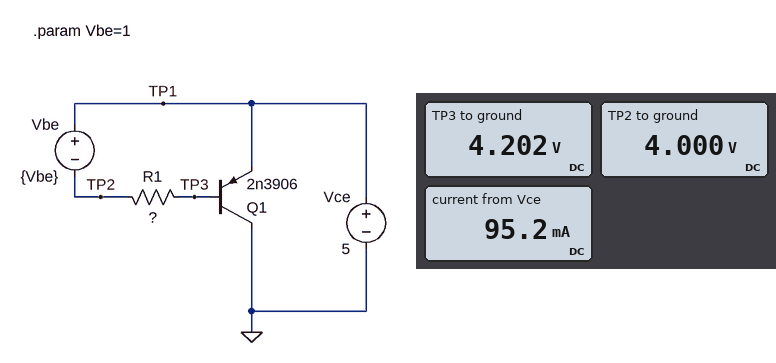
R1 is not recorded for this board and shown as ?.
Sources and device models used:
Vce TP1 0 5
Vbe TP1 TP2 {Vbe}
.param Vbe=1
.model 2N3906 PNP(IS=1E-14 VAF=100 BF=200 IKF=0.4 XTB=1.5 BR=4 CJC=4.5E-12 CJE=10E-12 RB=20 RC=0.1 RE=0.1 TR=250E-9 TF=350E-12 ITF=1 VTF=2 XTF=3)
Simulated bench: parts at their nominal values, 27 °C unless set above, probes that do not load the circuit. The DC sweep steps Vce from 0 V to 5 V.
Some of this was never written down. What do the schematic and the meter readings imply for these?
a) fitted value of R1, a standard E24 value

360 Ω
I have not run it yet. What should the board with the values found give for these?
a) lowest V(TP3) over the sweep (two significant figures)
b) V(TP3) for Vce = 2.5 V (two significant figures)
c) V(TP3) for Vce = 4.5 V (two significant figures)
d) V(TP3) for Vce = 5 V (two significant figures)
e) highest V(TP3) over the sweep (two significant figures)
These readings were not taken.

-700 mV
1.7 V
3.7 V
4.2 V
4.2 V
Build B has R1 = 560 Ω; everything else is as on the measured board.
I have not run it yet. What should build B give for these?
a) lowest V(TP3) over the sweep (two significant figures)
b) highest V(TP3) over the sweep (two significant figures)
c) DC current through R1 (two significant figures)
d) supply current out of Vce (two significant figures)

-690 mV
4.2 V
390 µA
69 mA
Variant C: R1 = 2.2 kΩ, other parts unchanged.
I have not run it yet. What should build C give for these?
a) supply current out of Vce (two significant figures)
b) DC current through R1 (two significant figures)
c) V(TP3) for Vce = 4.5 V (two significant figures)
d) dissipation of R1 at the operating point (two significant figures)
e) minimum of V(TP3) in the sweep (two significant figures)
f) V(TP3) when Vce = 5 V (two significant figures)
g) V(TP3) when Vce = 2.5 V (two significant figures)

23 mA
120 µA
3.8 V
30 µW
-650 mV
4.3 V
1.8 V
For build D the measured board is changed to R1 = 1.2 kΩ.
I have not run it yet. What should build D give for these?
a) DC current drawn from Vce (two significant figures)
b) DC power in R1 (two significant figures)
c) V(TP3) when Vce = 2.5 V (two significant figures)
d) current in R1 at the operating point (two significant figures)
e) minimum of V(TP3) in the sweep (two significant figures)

38 mA
49 µW
1.7 V
200 µA
-660 mV
